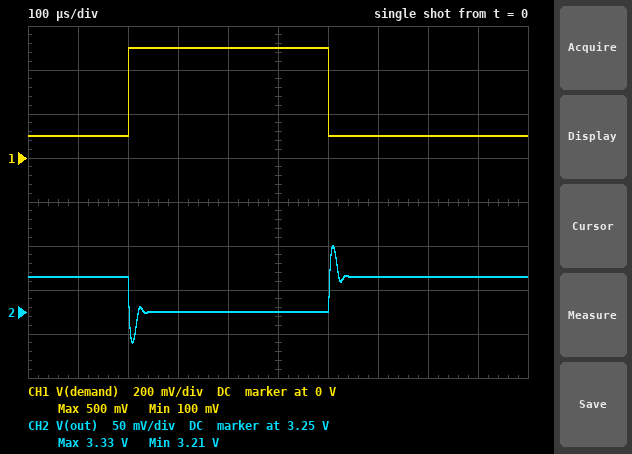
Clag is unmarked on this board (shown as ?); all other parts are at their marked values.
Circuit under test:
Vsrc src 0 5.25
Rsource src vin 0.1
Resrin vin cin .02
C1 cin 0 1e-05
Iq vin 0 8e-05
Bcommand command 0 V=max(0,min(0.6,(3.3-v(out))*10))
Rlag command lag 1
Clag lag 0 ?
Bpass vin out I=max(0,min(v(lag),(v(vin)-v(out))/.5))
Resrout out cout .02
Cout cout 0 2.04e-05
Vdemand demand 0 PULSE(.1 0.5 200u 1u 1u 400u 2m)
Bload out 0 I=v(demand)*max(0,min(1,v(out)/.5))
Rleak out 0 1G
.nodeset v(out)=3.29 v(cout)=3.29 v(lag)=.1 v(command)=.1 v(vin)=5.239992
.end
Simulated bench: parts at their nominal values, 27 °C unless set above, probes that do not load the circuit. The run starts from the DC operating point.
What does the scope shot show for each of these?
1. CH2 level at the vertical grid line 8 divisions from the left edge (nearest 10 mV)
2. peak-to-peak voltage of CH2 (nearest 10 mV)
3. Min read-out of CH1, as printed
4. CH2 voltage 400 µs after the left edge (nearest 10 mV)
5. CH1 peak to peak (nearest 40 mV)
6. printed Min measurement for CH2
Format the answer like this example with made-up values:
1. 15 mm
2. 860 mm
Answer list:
1. 3.29 V
2. 110 mV
3. 100 mV
4. 3.25 V
5. 400 mV
6. 3.21 V
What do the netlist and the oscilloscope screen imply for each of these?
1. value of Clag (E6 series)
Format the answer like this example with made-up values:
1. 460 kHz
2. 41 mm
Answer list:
1. 4.7 µF
